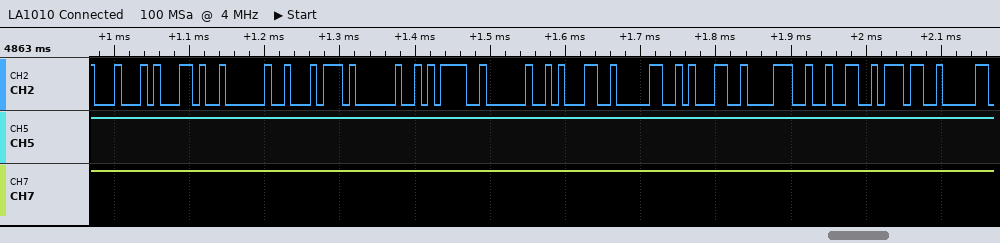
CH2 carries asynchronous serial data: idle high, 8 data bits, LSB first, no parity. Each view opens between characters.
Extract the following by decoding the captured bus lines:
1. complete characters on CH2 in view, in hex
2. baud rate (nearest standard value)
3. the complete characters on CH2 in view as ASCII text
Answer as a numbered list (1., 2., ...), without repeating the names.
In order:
1. 44, 2C, 20, 74, 20, 3D, 20, 31, 30, 31, 38, 32, 37
2. 115200 baud
3. "D, t = 101827"
